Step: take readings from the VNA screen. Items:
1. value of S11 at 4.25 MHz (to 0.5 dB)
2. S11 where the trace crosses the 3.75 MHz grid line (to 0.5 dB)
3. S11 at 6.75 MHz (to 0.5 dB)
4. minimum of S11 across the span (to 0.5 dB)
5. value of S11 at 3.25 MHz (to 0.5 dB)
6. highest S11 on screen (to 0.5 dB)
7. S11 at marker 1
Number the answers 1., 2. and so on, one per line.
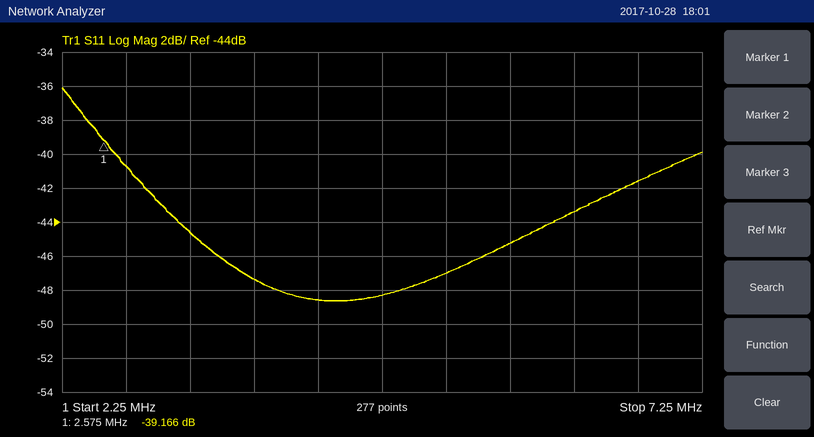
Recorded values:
1. -48.5 dB
2. -47.5 dB
3. -41.5 dB
4. -48.5 dB
5. -44.5 dB
6. -36.0 dB
7. -39.166 dB
